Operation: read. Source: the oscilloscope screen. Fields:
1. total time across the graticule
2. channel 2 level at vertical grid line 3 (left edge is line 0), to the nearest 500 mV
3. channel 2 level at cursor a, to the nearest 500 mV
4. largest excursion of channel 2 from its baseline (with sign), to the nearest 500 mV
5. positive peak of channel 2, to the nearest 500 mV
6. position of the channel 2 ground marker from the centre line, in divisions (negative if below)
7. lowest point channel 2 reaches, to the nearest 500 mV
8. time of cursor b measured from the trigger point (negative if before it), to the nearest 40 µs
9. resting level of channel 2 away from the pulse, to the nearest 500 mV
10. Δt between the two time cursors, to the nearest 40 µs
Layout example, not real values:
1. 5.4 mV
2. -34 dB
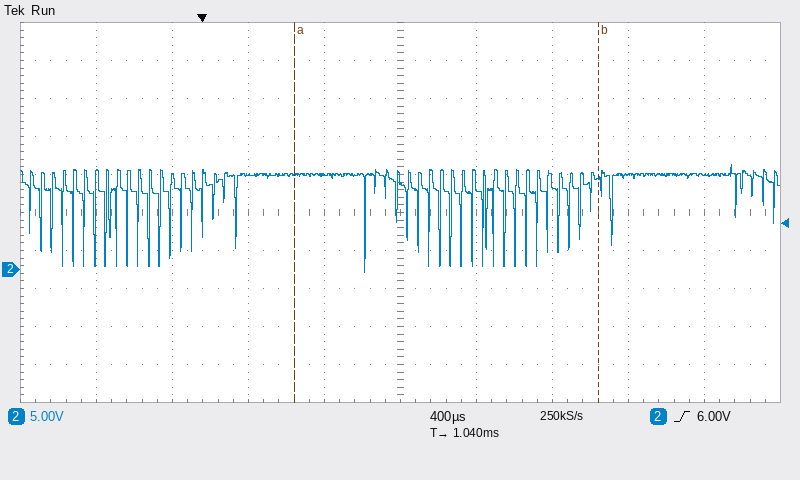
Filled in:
1. 4 ms
2. 12.5 V
3. 12.5 V
4. -13.0 V
5. 14.0 V
6. -1.5 div
7. -500 mV
8. +2.08 ms
9. 12.5 V
10. 1.60 ms
